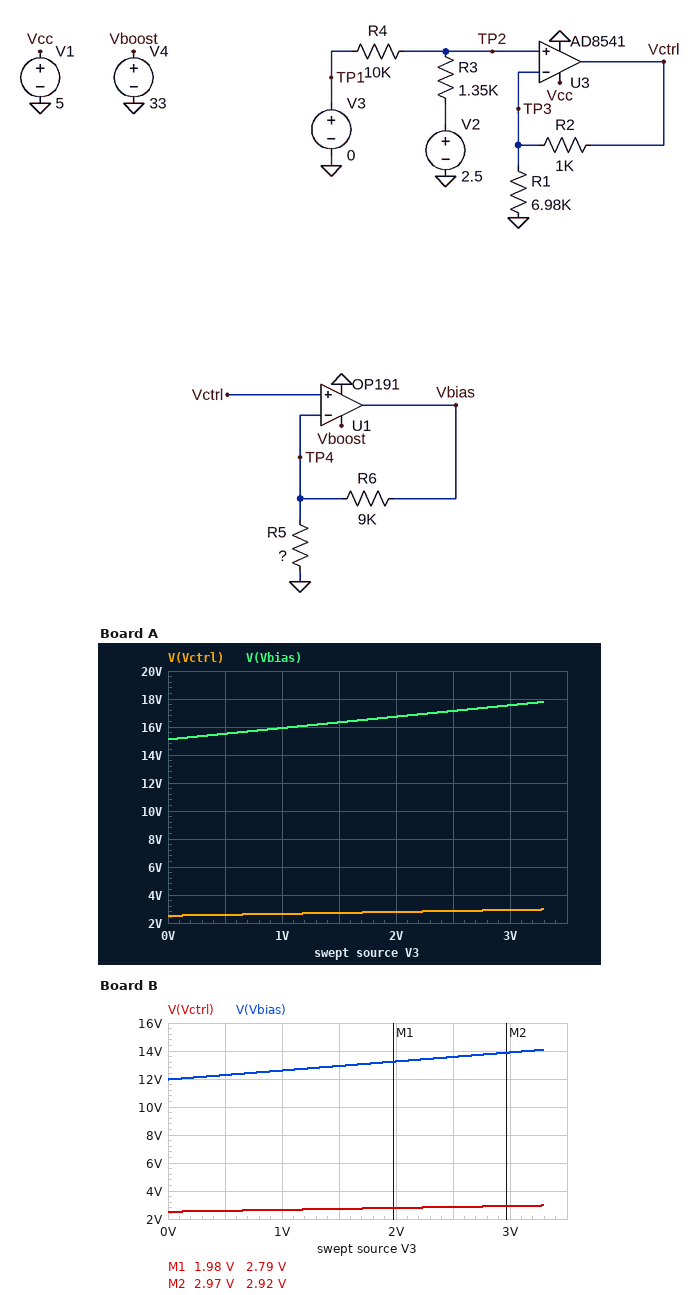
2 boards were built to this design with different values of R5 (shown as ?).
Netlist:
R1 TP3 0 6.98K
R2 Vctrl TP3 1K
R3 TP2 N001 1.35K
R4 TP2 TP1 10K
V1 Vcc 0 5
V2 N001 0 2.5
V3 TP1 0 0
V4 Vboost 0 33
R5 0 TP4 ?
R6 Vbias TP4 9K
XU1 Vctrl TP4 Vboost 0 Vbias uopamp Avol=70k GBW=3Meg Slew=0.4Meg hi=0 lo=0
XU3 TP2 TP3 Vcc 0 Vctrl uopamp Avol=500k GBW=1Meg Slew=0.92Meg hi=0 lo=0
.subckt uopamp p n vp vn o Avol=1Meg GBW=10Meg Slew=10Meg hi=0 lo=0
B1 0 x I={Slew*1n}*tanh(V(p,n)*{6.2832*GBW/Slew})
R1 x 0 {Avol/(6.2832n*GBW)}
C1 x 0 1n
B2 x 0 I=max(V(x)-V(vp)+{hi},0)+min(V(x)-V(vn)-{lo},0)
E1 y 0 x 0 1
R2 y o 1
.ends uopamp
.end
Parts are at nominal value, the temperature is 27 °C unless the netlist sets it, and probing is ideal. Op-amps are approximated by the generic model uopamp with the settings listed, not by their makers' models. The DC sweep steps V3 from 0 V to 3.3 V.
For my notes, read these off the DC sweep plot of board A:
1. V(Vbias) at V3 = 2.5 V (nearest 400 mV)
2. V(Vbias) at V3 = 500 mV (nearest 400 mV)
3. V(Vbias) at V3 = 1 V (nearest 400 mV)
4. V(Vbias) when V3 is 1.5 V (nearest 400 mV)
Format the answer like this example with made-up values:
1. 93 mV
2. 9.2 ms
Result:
1. 17.2 V
2. 15.6 V
3. 16.0 V
4. 16.4 V
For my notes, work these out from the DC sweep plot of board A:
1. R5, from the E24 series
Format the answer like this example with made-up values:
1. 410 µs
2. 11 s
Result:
1. 1.8 kΩ
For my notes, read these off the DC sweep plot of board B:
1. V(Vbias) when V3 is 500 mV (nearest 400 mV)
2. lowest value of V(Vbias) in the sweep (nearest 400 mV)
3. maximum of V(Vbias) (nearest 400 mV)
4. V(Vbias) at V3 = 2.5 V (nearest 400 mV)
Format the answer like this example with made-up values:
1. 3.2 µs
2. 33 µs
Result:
1. 12.4 V
2. 12.0 V
3. 14.0 V
4. 13.6 V
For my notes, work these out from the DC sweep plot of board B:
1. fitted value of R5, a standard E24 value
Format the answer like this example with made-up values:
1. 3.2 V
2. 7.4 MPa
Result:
1. 2.4 kΩ
